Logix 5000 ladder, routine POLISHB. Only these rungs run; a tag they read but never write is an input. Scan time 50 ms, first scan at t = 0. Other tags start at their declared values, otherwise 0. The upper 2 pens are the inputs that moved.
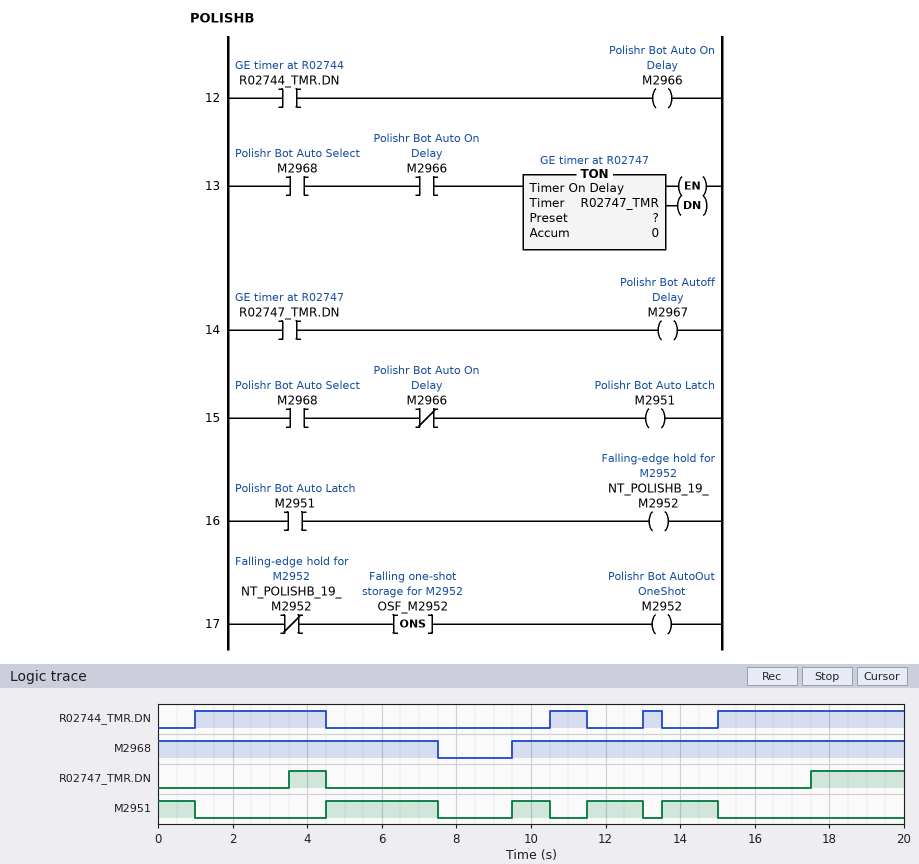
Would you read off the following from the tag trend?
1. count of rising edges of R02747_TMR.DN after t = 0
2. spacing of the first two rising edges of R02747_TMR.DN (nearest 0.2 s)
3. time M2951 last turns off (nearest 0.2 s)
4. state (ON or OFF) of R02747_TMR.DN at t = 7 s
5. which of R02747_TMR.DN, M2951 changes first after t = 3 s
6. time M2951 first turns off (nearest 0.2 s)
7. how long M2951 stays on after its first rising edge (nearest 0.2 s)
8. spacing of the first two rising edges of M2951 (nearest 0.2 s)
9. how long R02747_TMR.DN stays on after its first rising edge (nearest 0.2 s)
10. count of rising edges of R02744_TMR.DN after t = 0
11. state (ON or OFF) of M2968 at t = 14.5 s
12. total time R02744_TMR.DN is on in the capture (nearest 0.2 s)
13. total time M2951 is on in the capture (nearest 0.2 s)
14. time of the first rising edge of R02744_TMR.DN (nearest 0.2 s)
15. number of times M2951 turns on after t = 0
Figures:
2
14.0 s
15.0 s
OFF
R02747_TMR.DN
1.0 s
3.0 s
5.0 s
1.0 s
4
ON
10.0 s
8.0 s
1.0 s
4
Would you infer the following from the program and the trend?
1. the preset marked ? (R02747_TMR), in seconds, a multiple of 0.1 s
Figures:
2.5 s
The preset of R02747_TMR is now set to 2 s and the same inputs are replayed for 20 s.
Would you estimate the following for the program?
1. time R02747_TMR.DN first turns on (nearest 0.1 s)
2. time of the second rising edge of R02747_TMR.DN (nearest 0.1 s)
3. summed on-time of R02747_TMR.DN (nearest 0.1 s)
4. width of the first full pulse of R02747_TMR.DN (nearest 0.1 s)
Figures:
3.0 s
17.0 s
4.5 s
1.5 s
